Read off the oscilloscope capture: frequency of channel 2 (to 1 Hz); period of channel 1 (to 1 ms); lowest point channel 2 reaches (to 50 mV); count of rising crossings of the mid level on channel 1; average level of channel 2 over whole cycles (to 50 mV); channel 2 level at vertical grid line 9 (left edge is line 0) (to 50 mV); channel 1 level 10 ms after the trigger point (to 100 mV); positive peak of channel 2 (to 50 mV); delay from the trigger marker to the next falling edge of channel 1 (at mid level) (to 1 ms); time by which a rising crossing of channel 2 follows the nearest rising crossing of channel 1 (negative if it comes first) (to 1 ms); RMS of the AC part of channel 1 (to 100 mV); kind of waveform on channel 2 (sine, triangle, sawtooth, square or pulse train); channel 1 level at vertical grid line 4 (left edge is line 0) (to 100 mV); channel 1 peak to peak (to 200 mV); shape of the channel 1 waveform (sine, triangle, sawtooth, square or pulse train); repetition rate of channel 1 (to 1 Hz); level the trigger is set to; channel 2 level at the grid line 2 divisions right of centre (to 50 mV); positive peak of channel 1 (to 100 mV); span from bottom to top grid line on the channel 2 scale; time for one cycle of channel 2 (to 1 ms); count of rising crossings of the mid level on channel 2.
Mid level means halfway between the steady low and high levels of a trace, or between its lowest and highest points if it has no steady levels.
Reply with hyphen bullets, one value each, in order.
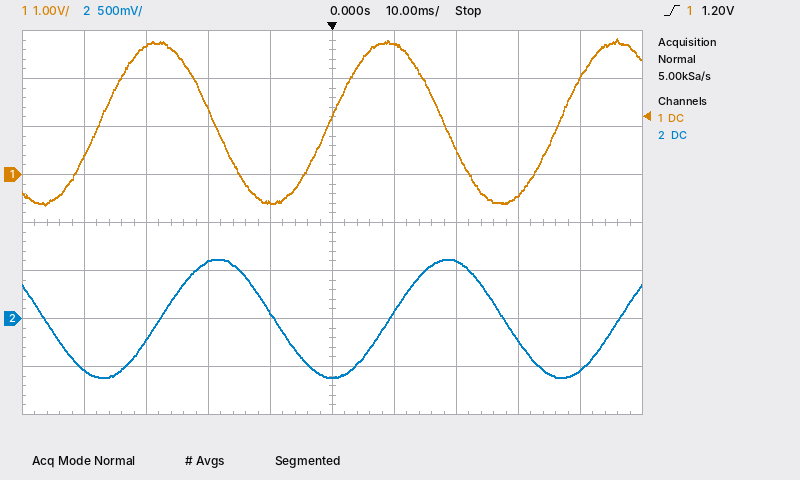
- 27 Hz
- 37 ms
- -600 mV
- 3
- 0 mV
- -550 mV
- 2.7 V
- 600 mV
- 18 ms
- +10 ms
- 1.2 V
- sine
- -600 mV
- 3.4 V
- sine
- 27 Hz
- 1.20 V
- 600 mV
- 2.8 V
- 4 V
- 37 ms
- 3
